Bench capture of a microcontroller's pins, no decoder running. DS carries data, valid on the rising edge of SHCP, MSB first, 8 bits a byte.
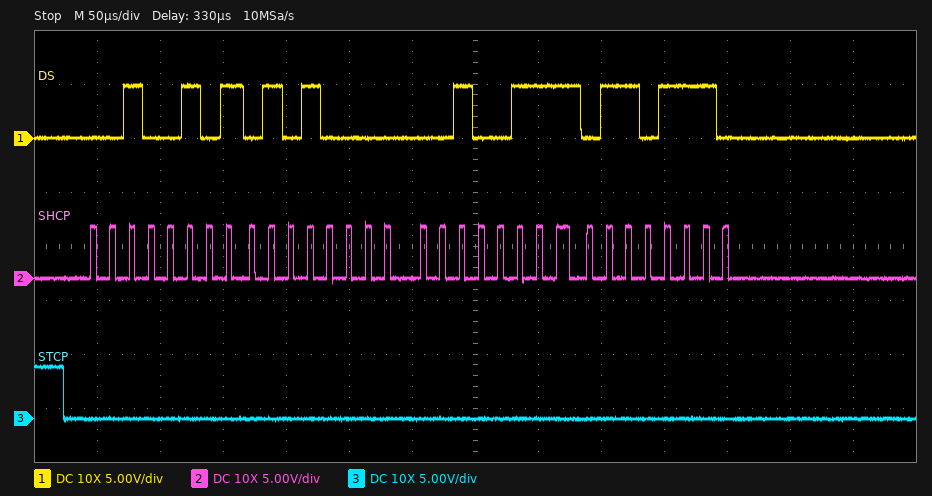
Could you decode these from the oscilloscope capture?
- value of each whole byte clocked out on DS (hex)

25 50 27 6E
